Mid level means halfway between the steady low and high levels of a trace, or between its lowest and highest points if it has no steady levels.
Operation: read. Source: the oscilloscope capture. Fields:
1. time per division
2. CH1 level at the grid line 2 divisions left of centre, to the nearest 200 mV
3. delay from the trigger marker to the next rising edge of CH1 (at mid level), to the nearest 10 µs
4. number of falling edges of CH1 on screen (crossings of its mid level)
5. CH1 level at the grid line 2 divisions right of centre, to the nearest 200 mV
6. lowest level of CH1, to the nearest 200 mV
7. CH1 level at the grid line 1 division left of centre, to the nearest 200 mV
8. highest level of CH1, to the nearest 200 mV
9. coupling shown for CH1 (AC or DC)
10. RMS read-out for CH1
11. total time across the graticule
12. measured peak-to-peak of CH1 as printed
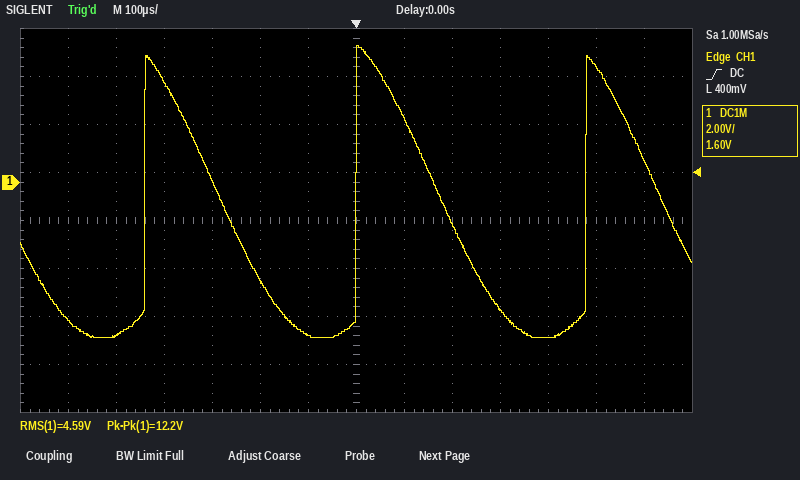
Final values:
100 µs
-4.0 V
480 µs
3
-1.8 V
-6.4 V
-6.4 V
5.6 V
DC
4.59 V
1.4 ms
12.2 V
